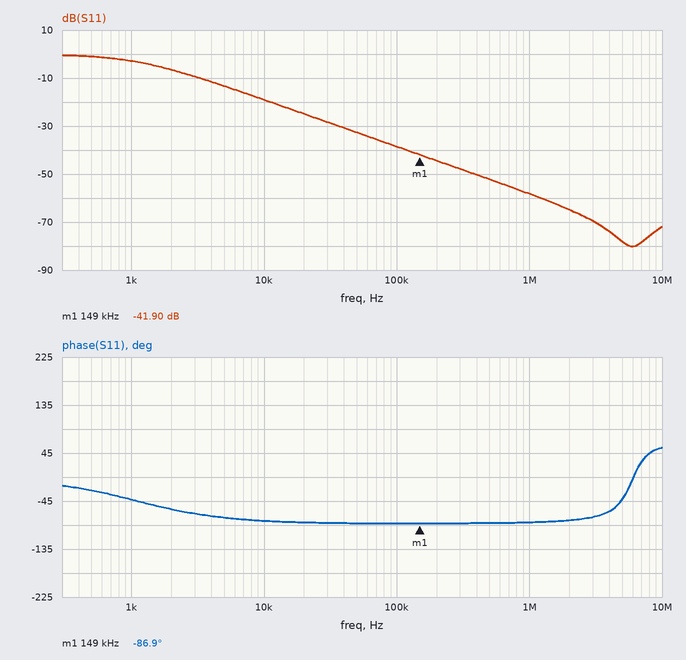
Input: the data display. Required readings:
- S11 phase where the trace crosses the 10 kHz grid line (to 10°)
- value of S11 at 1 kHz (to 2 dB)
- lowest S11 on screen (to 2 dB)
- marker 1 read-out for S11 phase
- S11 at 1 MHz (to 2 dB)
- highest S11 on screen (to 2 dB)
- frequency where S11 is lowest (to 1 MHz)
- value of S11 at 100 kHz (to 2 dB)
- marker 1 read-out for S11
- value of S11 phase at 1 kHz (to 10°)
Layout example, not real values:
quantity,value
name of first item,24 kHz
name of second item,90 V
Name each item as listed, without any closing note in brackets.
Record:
quantity,value
S11 phase where the trace crosses the 10 kHz grid line,-80°
value of S11 at 1 kHz,-2 dB
lowest S11 on screen,-80 dB
marker 1 read-out for S11 phase,-86.9°
S11 at 1 MHz,-58 dB
highest S11 on screen,0 dB
frequency where S11 is lowest,6 MHz
value of S11 at 100 kHz,-38 dB
marker 1 read-out for S11,-41.90 dB
value of S11 phase at 1 kHz,-40°
